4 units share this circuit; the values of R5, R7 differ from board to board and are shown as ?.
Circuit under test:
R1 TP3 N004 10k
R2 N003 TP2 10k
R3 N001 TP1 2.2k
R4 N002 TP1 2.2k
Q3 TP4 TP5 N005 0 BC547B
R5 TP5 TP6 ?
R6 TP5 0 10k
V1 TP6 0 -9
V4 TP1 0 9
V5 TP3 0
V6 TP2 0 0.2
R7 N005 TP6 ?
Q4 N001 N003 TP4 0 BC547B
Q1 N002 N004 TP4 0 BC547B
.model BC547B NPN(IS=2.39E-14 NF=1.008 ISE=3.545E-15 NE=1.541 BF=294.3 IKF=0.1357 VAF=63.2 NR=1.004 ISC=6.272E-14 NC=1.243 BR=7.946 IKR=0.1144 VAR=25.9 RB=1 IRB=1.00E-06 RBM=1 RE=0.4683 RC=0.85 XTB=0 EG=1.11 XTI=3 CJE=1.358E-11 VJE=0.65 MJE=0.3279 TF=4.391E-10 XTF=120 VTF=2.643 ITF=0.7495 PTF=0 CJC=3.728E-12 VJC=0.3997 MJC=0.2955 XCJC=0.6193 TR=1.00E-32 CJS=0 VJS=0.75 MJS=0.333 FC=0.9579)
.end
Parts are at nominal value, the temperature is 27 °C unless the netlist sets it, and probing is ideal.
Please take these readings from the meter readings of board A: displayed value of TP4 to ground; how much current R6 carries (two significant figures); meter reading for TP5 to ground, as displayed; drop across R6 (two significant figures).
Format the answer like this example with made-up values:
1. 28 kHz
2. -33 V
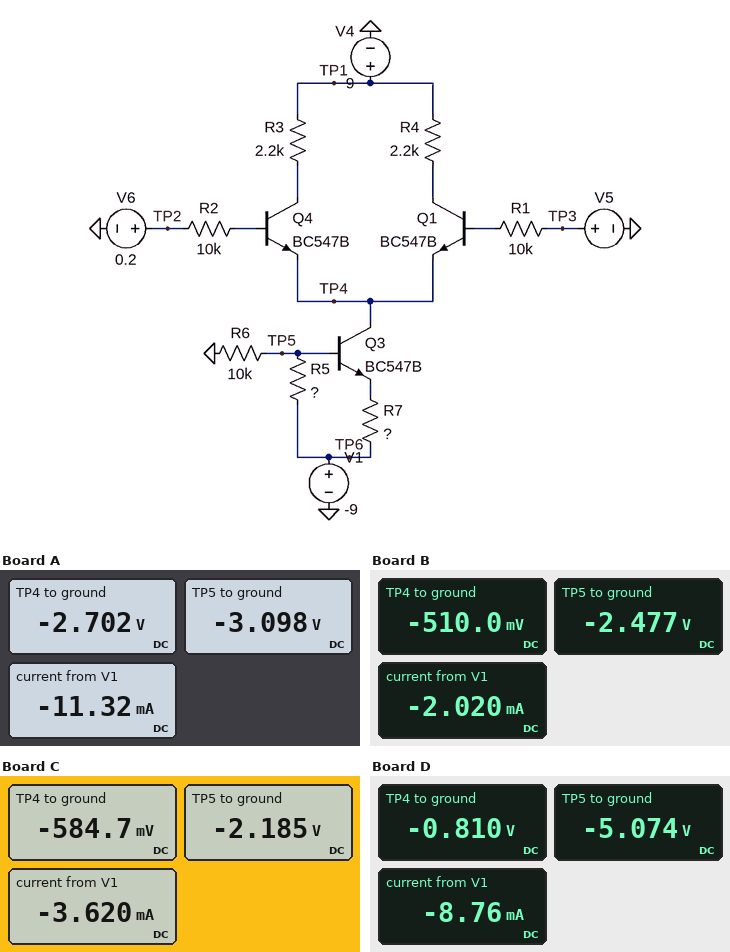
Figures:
1. -2.702 V
2. 310 µA
3. -3.098 V
4. 3.1 V
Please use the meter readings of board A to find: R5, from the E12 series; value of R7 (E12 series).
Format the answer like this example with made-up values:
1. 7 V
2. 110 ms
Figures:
1. 22 kΩ
2. 470 Ω
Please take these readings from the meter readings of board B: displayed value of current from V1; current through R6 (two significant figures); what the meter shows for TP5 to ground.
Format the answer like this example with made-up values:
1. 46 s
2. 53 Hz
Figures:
1. -2.020 mA
2. 250 µA
3. -2.477 V
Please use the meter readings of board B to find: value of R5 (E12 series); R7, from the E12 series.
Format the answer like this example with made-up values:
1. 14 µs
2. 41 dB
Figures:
1. 27 kΩ
2. 3.3 kΩ
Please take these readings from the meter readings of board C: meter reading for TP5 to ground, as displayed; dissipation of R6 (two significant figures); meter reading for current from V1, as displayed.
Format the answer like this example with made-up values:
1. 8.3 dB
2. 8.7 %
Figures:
1. -2.185 V
2. 480 µW
3. -3.620 mA
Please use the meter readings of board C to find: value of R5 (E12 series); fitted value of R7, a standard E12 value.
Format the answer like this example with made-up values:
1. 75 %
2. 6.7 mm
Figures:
1. 33 kΩ
2. 1.8 kΩ
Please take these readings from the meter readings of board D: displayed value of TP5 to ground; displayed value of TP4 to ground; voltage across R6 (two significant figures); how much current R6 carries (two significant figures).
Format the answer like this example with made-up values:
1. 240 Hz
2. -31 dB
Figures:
1. -5.074 V
2. -0.810 V
3. 5.1 V
4. 510 µA
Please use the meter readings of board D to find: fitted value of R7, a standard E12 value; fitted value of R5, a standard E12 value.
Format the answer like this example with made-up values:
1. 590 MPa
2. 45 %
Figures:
1. 390 Ω
2. 8.2 kΩ
